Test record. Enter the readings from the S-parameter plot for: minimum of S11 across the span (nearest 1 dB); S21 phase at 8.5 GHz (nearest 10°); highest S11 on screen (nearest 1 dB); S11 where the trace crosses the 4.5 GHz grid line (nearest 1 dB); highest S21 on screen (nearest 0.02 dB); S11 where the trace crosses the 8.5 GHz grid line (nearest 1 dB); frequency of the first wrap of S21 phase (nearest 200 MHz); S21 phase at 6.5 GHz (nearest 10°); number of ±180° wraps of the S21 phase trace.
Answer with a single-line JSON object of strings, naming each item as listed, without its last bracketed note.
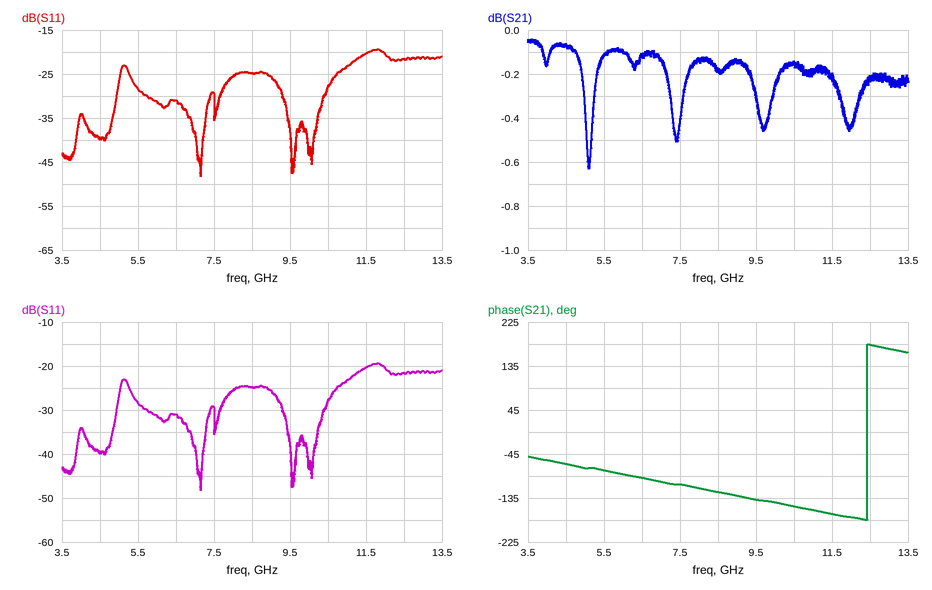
{"minimum of S11 across the span": "-48 dB", "S21 phase at 8.5 GHz": "-120°", "highest S11 on screen": "-19 dB", "S11 where the trace crosses the 4.5 GHz grid line": "-40 dB", "highest S21 on screen": "-0.04 dB", "S11 where the trace crosses the 8.5 GHz grid line": "-25 dB", "frequency of the first wrap of S21 phase": "12.4 GHz", "S21 phase at 6.5 GHz": "-90°", "number of ±180° wraps of the S21 phase trace": "1"}
